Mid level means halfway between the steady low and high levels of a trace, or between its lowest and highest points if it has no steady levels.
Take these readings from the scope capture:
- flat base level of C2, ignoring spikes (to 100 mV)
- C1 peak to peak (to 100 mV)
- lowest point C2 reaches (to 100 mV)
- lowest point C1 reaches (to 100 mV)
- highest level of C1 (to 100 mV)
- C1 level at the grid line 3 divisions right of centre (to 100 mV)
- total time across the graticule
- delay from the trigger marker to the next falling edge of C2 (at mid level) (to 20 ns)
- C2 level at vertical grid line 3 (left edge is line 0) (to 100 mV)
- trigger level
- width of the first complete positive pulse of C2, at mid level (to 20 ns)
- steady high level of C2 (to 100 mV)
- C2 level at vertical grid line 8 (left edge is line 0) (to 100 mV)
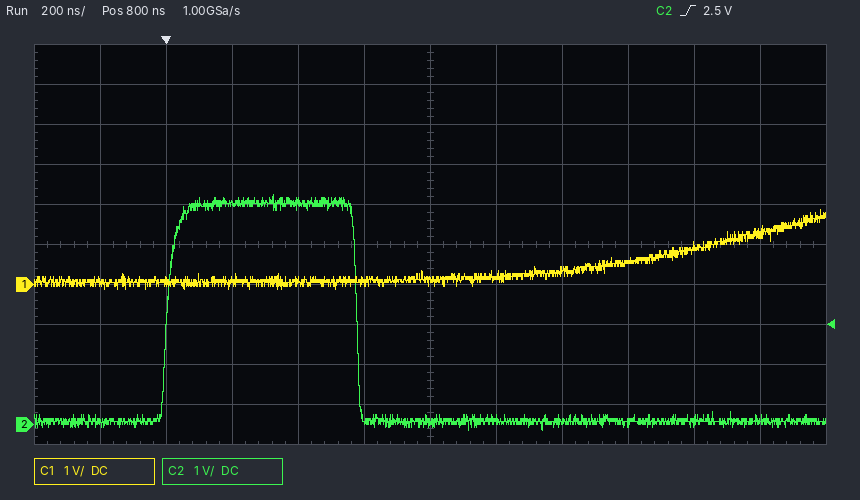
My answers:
100 mV
2.0 V
-200 mV
-100 mV
1.9 V
600 mV
2.4 µs
580 ns
5.5 V
2.5 V
580 ns
5.5 V
100 mV
